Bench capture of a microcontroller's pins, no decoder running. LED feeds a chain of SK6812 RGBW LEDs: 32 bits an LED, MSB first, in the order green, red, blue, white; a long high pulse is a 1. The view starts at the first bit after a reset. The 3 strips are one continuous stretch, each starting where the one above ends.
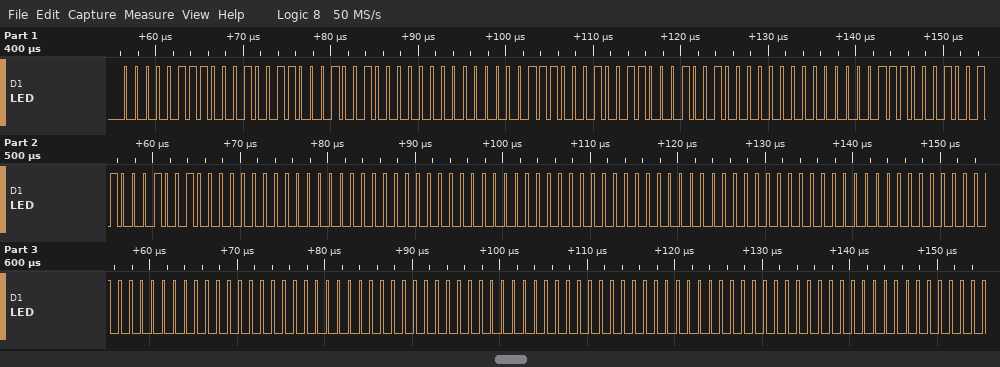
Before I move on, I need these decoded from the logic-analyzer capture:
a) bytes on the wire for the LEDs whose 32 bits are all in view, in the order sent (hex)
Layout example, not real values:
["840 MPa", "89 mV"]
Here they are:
["07 13 12 00 07 13 12 00 07 13 12 00 00 00 00 00 00 00 00 00 00 00 00 00 00 00 00 00"]
